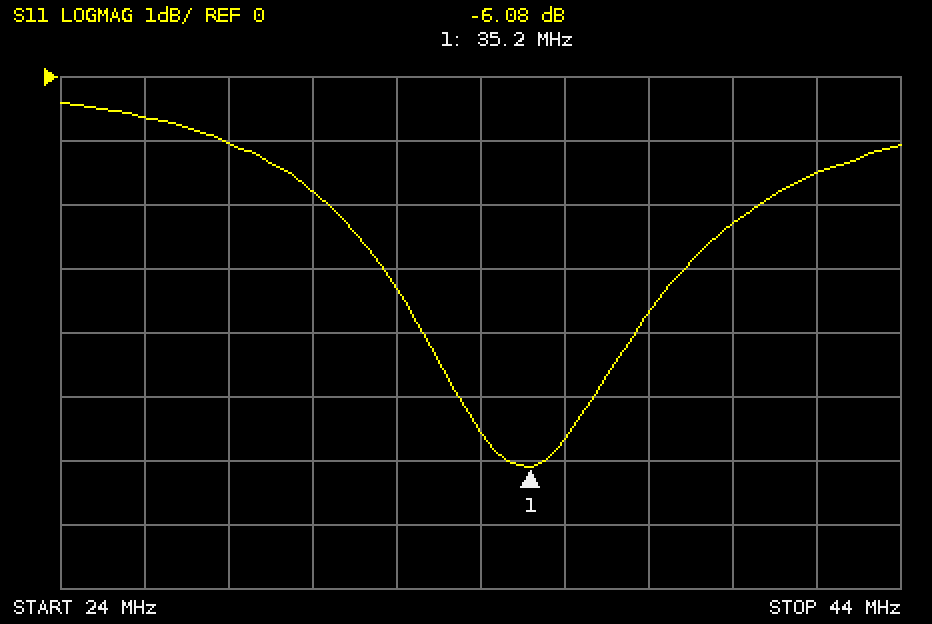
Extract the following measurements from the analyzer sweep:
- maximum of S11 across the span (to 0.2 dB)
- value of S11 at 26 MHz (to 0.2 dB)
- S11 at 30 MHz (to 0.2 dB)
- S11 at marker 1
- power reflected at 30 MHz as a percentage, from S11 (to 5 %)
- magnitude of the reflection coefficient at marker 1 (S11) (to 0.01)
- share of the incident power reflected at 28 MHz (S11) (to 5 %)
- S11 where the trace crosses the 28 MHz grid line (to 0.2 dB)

-0.4 dB
-0.6 dB
-1.8 dB
-6.08 dB
65 %
0.50
80 %
-1.0 dB
